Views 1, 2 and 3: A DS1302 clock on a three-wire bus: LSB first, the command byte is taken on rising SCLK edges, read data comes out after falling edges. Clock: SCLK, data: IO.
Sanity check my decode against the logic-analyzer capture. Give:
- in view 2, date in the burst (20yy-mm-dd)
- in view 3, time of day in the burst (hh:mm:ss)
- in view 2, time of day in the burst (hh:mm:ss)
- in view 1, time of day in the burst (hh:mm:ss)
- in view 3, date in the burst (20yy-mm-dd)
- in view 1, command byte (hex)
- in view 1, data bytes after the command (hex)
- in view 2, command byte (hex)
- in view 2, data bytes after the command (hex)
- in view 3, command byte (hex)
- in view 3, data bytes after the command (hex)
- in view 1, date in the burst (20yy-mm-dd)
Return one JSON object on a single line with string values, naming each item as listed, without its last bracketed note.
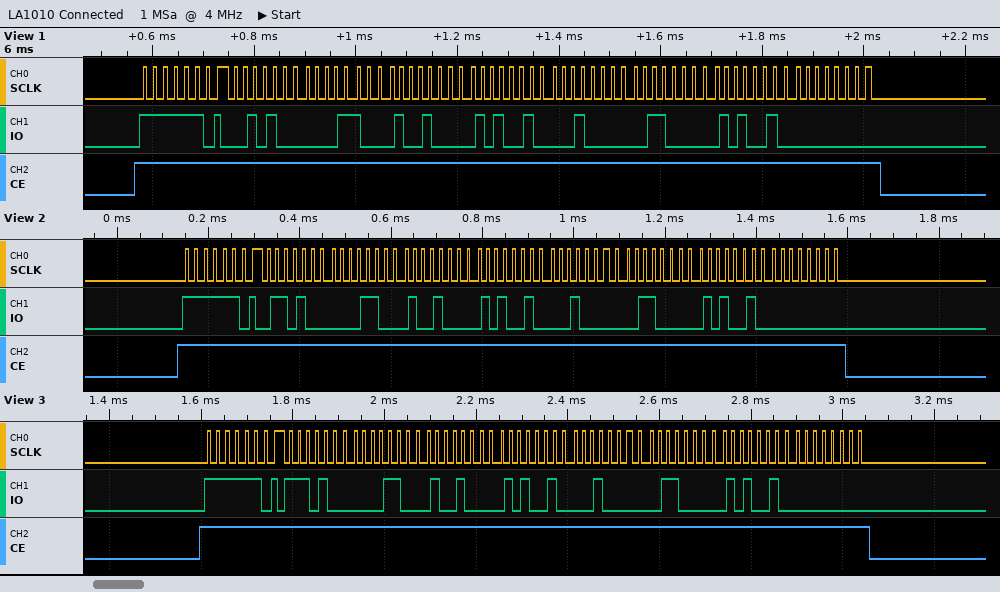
{"in view 2, date in the burst": "2025-04-25", "in view 3, time of day in the burst": "09:18:17", "in view 2, time of day in the burst": "09:18:16", "in view 1, time of day in the burst": "09:18:14", "in view 3, date in the burst": "2025-04-25", "in view 1, command byte": "0xBF", "in view 1, data bytes after the command": "14 18 09 25 04 06 25 00", "in view 2, command byte": "0xBF", "in view 2, data bytes after the command": "16 18 09 25 04 06 25 00", "in view 3, command byte": "0xBF", "in view 3, data bytes after the command": "17 18 09 25 04 06 25 00", "in view 1, date in the burst": "2025-04-25"}
